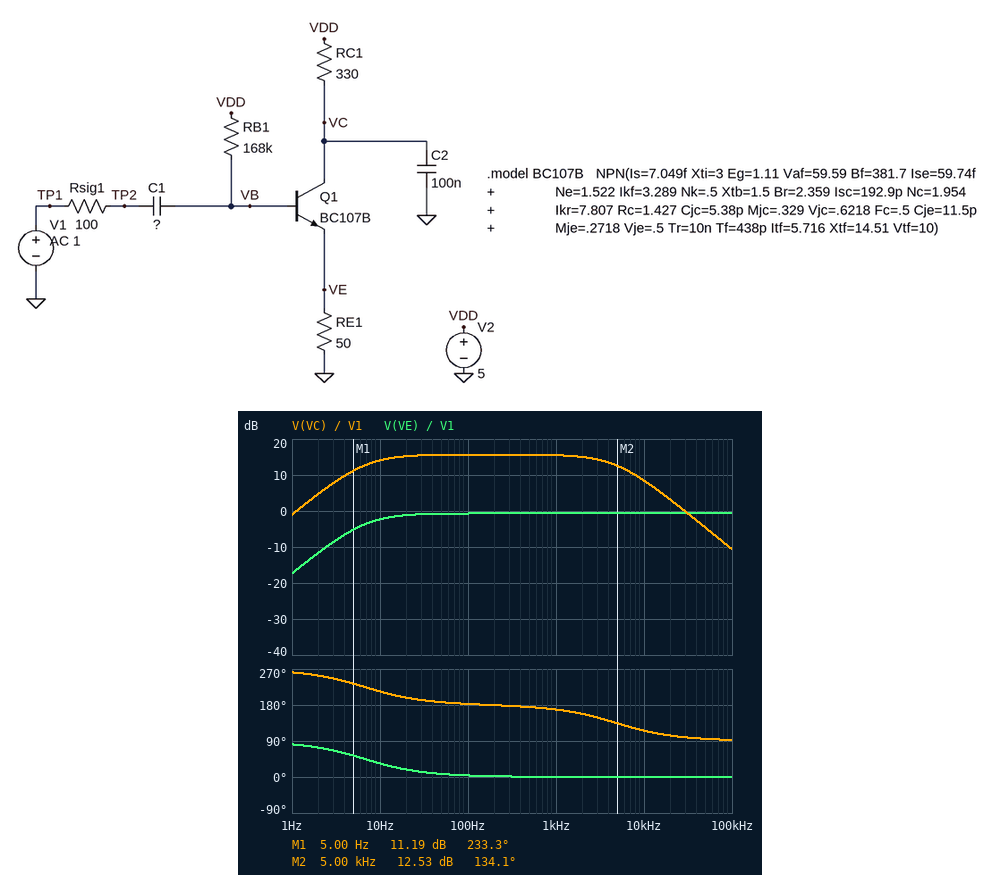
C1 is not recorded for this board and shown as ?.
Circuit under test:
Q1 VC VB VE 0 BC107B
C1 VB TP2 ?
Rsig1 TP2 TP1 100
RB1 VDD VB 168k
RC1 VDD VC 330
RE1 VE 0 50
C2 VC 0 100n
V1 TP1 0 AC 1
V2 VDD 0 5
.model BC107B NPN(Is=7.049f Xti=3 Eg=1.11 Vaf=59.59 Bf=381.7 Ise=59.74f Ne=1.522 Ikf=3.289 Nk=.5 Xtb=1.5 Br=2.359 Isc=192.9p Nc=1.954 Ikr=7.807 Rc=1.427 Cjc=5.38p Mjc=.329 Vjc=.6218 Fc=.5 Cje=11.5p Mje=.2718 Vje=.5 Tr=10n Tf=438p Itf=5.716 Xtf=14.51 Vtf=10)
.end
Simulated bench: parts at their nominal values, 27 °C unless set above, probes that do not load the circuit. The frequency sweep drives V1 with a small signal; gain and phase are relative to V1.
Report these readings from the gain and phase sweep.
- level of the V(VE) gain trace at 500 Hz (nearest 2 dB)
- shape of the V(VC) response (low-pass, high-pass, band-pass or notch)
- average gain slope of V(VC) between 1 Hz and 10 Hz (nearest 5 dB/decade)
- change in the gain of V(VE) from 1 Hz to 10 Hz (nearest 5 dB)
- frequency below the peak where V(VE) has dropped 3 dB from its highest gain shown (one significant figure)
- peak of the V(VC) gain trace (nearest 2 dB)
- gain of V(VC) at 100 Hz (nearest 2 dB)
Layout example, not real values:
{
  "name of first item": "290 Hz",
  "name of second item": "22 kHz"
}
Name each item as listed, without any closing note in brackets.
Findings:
{
  "level of the V(VE) gain trace at 500 Hz": "0 dB",
  "shape of the V(VC) response": "band-pass",
  "average gain slope of V(VC) between 1 Hz and 10 Hz": "15 dB/decade",
  "change in the gain of V(VE) from 1 Hz to 10 Hz": "15 dB",
  "frequency below the peak where V(VE) has dropped 3 dB from its highest gain shown": "7 Hz",
  "peak of the V(VC) gain trace": "16 dB",
  "gain of V(VC) at 100 Hz": "16 dB"
}
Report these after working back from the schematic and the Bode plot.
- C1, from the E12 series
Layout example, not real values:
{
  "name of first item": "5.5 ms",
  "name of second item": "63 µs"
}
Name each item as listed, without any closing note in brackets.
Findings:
{
  "C1, from the E12 series": "1.5 µF"
}
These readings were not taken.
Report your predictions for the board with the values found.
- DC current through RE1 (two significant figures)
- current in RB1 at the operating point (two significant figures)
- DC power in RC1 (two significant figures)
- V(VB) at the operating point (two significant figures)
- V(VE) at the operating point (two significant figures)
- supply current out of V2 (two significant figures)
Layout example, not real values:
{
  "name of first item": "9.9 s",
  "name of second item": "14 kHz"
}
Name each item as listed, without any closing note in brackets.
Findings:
{
  "DC current through RE1": "7.3 mA",
  "current in RB1 at the operating point": "23 µA",
  "DC power in RC1": "18 mW",
  "V(VB) at the operating point": "1.1 V",
  "V(VE) at the operating point": "370 mV",
  "supply current out of V2": "7.3 mA"
}
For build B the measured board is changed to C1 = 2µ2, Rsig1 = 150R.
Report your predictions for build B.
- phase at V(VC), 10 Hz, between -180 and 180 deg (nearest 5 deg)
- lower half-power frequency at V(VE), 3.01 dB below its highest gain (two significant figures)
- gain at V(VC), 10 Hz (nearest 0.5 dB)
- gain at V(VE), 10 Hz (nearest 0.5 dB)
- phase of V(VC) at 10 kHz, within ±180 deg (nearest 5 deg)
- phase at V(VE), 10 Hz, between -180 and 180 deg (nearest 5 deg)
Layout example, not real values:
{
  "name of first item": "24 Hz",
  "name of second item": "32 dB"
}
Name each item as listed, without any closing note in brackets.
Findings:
{
  "phase at V(VC), 10 Hz, between -180 and 180 deg": "-155 deg",
  "lower half-power frequency at V(VE), 3.01 dB below its highest gain": "4.6 Hz",
  "gain at V(VC), 10 Hz": "15.0 dB",
  "gain at V(VE), 10 Hz": "-1.5 dB",
  "phase of V(VC) at 10 kHz, within ±180 deg": "115 deg",
  "phase at V(VE), 10 Hz, between -180 and 180 deg": "25 deg"
}
